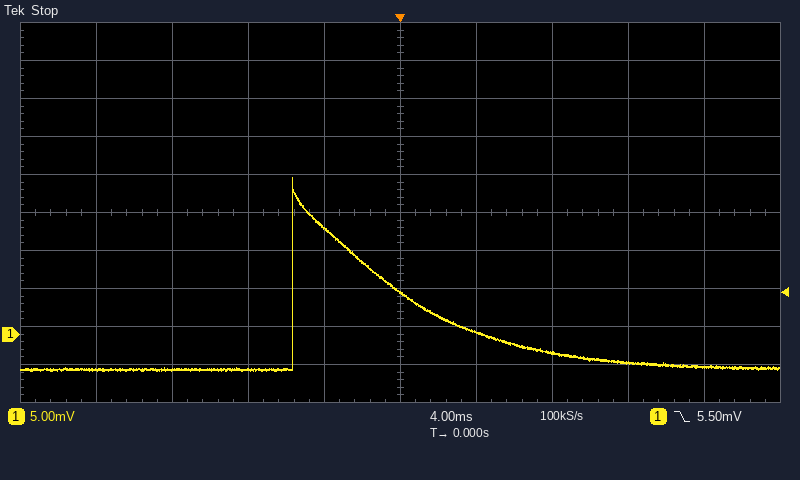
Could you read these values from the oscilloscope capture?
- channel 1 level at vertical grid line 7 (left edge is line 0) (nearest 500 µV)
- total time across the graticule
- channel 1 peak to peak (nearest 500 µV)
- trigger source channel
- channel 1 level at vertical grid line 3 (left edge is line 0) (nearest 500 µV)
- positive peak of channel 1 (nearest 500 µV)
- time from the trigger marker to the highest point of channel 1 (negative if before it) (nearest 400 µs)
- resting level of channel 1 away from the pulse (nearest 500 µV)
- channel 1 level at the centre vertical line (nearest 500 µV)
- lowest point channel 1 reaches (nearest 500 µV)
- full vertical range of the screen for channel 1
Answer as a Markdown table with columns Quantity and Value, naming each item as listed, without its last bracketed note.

| Quantity | Value |
|---|---|
| channel 1 level at vertical grid line 7 (left edge is line 0) | -2.5 mV |
| total time across the graticule | 40 ms |
| channel 1 peak to peak | 25.5 mV |
| trigger source channel | channel 1 |
| channel 1 level at vertical grid line 3 (left edge is line 0) | -4.5 mV |
| positive peak of channel 1 | 20.5 mV |
| time from the trigger marker to the highest point of channel 1 (negative if before it) | -5.6 ms |
| resting level of channel 1 away from the pulse | -4.5 mV |
| channel 1 level at the centre vertical line | 5.5 mV |
| lowest point channel 1 reaches | -5.0 mV |
| full vertical range of the screen for channel 1 | 50 mV |
